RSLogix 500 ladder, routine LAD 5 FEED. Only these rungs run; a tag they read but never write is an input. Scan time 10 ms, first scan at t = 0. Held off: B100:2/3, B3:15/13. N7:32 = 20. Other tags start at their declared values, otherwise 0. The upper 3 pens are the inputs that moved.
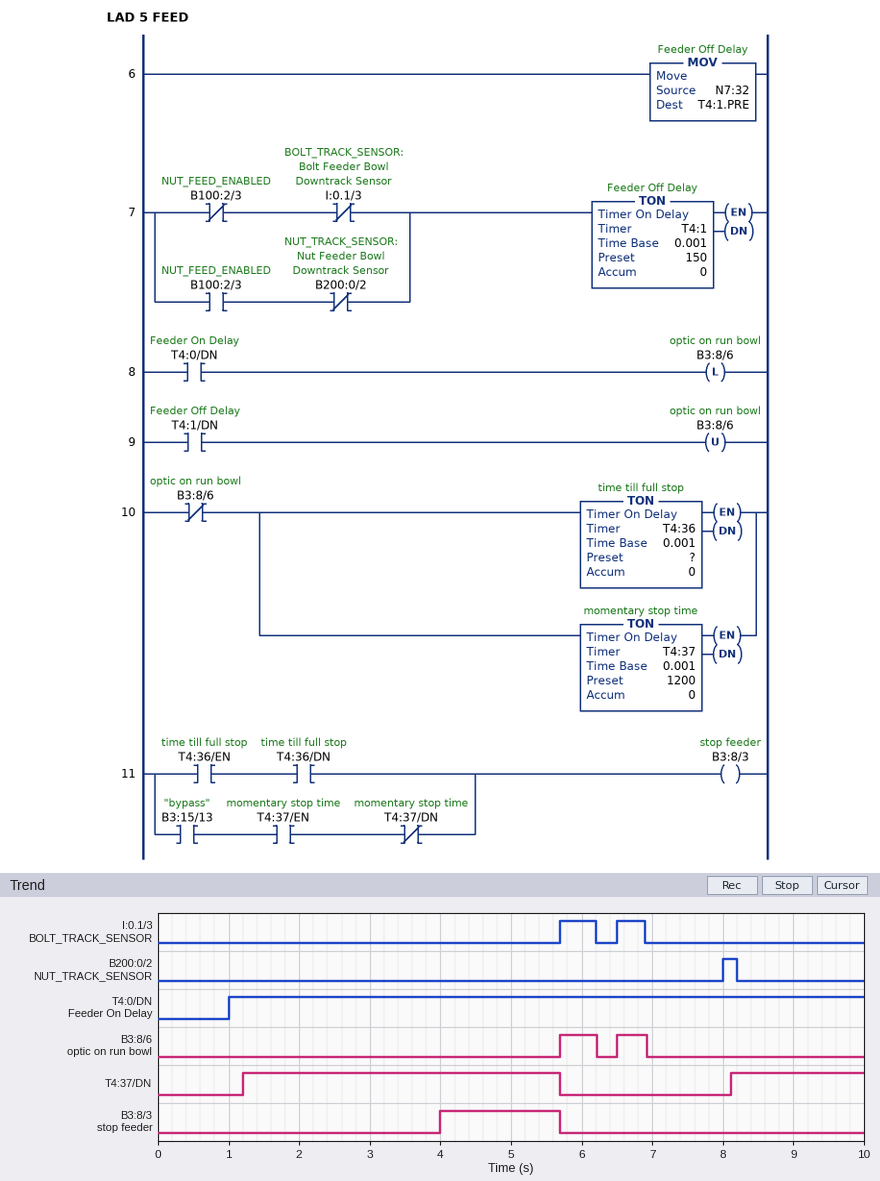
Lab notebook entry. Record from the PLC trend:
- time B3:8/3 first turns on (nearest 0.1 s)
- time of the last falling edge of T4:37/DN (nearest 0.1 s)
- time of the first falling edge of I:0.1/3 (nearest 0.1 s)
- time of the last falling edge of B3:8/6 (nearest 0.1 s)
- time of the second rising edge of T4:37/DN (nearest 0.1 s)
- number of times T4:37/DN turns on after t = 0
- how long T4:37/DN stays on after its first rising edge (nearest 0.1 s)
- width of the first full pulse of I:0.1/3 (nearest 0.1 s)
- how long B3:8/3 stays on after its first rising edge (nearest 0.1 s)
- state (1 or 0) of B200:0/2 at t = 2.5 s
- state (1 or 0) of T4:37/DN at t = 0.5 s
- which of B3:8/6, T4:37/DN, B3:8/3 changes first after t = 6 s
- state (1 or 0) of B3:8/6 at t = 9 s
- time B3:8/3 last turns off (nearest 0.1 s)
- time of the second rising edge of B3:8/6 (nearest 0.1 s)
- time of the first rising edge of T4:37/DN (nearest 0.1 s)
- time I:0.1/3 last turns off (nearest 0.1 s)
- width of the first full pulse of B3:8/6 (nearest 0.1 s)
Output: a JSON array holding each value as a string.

["4.0 s", "5.7 s", "6.2 s", "6.9 s", "8.1 s", "2", "4.5 s", "0.5 s", "1.7 s", "0", "0", "B3:8/6", "0", "5.7 s", "6.5 s", "1.2 s", "6.9 s", "0.5 s"]
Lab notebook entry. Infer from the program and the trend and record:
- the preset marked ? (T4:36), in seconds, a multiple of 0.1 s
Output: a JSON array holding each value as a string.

["4.0 s"]
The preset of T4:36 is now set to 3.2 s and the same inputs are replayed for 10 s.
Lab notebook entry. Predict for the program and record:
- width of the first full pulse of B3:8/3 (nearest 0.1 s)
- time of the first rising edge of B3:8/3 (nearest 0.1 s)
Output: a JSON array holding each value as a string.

["2.5 s", "3.2 s"]
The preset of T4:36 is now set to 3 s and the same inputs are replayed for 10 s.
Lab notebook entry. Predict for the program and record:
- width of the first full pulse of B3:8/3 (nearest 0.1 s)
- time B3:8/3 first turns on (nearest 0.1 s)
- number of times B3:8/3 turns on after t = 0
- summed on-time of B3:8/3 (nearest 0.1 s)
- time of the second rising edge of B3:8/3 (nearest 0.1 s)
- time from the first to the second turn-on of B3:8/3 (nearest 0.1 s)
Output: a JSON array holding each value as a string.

["2.7 s", "3.0 s", "2", "2.8 s", "9.9 s", "6.9 s"]
